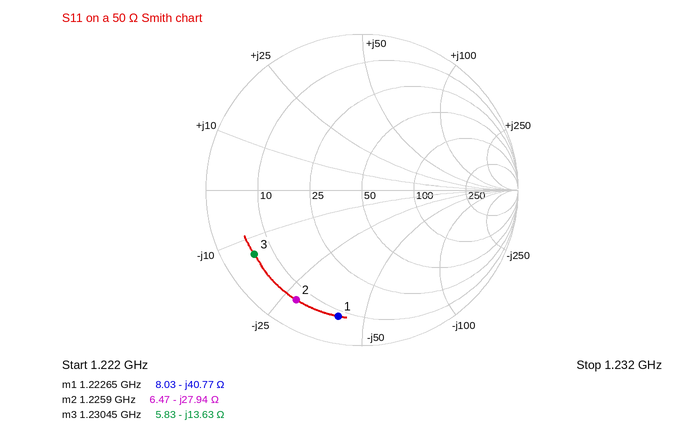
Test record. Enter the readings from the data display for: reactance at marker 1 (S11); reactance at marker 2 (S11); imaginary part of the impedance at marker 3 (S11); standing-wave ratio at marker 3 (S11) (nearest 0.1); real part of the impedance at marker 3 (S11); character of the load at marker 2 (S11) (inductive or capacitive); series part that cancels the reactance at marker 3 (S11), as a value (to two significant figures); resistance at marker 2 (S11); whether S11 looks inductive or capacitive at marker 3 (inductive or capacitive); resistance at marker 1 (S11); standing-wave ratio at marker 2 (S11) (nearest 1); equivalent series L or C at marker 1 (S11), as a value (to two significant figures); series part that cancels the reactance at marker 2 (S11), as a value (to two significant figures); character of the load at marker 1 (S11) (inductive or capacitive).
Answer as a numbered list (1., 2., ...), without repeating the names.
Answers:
1. -40.77 Ω
2. -27.94 Ω
3. -13.63 Ω
4. 9.2
5. 5.83 Ω
6. capacitive
7. 1.8 nH
8. 6.47 Ω
9. capacitive
10. 8.03 Ω
11. 10
12. 3.2 pF
13. 3.6 nH
14. capacitive
